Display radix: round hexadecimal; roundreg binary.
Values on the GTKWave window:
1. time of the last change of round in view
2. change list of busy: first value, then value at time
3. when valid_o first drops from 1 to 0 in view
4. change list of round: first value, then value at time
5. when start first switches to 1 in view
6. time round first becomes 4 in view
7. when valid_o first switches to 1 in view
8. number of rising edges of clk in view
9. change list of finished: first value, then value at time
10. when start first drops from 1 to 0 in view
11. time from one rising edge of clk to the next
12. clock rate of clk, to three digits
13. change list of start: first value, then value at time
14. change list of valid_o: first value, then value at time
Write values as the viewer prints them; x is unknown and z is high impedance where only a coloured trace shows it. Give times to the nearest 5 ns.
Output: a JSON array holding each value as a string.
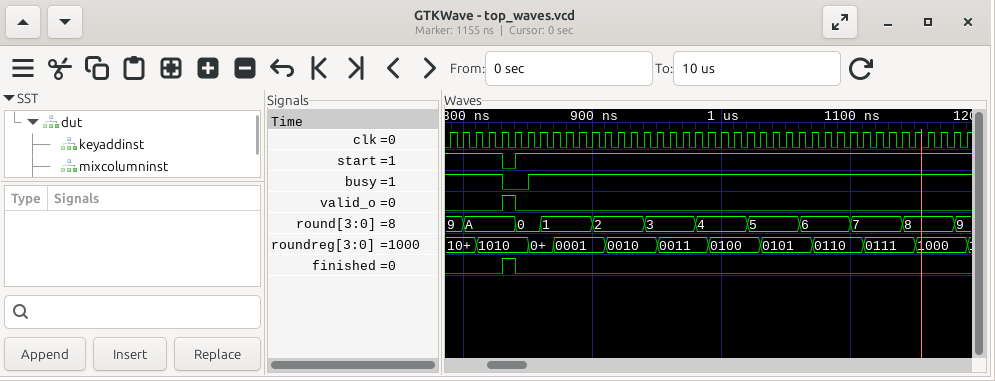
["1180 ns", "1, 0 at 830 ns, 1 at 850 ns", "840 ns", "9, A at 800 ns, 0 at 840 ns, 1 at 860 ns, 2 at 900 ns, 3 at 940 ns, 4 at 980 ns, 5 at 1020 ns, 6 at 1060 ns, 7 at 1100 ns, 8 at 1140 ns, 9 at 1180 ns", "840 ns", "980 ns", "830 ns", "41", "0, 1 at 830 ns, 0 at 840 ns", "830 ns", "10 ns", "100 MHz", "1, 0 at 830 ns, 1 at 840 ns", "0, 1 at 830 ns, 0 at 840 ns"]
